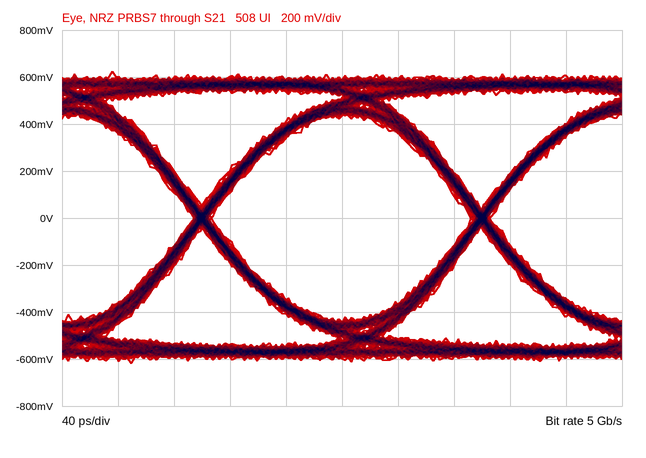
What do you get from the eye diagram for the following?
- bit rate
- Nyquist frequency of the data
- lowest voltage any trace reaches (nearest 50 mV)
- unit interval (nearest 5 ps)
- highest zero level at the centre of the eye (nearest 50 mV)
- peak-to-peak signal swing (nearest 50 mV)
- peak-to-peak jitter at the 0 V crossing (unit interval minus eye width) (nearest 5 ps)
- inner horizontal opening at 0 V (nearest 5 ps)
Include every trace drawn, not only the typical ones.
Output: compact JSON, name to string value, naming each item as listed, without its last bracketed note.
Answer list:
{"bit rate": "5 Gb/s", "Nyquist frequency of the data": "2.5 GHz", "lowest voltage any trace reaches": "-600 mV", "unit interval": "200 ps", "highest zero level at the centre of the eye": "-450 mV", "peak-to-peak signal swing": "1.25 V", "peak-to-peak jitter at the 0 V crossing (unit interval minus eye width)": "15 ps", "inner horizontal opening at 0 V": "185 ps"}
